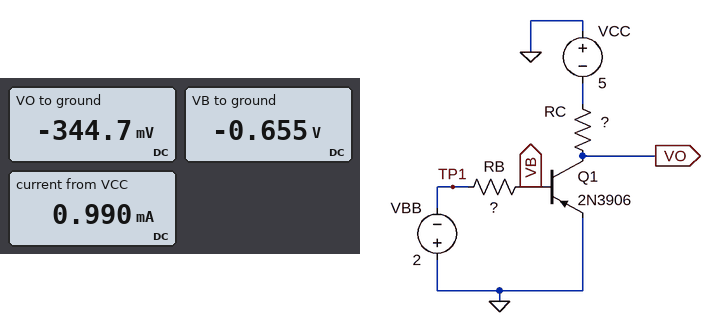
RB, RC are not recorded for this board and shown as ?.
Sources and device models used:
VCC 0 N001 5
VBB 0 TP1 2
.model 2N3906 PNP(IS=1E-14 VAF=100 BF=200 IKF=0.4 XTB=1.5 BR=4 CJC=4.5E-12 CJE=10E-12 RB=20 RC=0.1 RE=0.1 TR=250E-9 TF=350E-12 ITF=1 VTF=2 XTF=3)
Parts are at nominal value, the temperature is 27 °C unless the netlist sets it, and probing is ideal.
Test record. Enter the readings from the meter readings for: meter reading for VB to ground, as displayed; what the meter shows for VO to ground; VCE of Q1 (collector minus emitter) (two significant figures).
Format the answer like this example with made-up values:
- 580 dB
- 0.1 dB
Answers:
- -0.655 V
- -344.7 mV
- -340 mV
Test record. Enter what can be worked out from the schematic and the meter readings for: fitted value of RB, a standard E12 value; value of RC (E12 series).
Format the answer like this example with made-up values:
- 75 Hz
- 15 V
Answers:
- 270 kΩ
- 4.7 kΩ
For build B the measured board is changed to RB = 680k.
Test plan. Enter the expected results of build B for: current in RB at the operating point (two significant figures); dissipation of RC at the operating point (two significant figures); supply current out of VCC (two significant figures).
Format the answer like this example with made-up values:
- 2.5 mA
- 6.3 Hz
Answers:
- 2.0 µA
- 800 µW
- 410 µA
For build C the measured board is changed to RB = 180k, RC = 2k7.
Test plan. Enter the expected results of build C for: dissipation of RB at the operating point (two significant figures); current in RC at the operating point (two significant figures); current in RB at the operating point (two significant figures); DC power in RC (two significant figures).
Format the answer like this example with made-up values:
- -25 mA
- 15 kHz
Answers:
- 9.9 µW
- 1.5 mA
- 7.4 µA
- 5.9 mW
